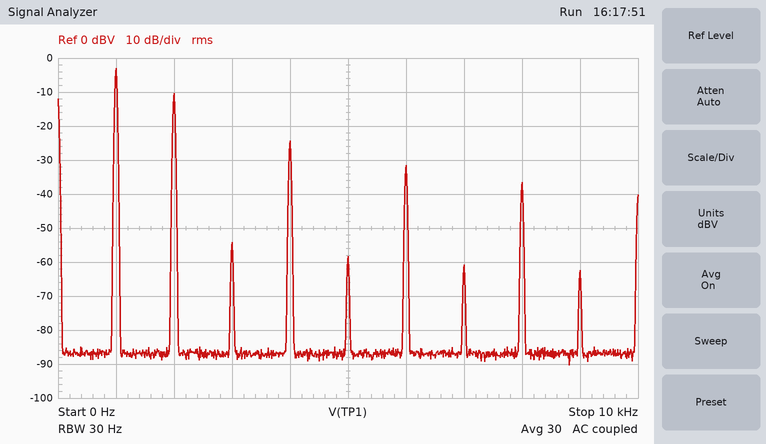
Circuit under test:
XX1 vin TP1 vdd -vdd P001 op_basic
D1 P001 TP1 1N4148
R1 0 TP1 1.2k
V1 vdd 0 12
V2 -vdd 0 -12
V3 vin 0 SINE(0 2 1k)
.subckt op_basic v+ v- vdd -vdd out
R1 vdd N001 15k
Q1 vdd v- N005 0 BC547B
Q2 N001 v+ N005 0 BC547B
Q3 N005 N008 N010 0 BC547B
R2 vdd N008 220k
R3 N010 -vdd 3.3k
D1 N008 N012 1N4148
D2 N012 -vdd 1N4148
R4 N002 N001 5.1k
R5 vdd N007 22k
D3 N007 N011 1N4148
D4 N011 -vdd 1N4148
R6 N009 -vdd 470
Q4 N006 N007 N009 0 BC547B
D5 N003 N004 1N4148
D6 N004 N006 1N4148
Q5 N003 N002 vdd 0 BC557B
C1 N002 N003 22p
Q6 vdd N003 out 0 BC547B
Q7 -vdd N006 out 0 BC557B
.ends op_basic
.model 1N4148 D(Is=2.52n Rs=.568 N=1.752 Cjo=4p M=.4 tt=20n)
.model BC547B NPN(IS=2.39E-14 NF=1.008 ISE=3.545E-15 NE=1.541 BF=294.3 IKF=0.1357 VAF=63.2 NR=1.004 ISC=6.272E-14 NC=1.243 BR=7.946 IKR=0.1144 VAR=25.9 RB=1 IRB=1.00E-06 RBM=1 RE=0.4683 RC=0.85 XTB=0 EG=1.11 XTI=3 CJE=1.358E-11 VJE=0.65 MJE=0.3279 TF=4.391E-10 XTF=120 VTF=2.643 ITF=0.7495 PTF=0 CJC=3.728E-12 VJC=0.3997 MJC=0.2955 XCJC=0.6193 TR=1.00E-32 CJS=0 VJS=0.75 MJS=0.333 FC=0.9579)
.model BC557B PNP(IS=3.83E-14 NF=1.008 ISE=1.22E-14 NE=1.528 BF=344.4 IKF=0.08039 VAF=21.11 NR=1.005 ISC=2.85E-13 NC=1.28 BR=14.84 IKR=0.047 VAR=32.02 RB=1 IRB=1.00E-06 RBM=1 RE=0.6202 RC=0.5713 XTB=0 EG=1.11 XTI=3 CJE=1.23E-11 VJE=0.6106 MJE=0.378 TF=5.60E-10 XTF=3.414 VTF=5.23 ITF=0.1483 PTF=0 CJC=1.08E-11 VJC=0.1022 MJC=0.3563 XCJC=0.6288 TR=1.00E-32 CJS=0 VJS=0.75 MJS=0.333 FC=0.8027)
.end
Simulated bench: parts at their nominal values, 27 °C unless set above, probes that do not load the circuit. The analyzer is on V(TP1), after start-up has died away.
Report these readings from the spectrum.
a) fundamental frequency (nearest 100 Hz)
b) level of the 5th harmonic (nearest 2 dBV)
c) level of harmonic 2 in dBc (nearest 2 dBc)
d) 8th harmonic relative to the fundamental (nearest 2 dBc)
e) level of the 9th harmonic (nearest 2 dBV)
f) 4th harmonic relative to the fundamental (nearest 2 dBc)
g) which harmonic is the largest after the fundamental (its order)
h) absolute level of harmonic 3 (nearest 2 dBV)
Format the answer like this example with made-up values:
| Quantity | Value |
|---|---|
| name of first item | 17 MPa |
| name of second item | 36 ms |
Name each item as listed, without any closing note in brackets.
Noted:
| Quantity | Value |
|---|---|
| fundamental frequency | 1.0 kHz |
| level of the 5th harmonic | -58 dBV |
| level of harmonic 2 in dBc | -8 dBc |
| 8th harmonic relative to the fundamental | -34 dBc |
| level of the 9th harmonic | -62 dBV |
| 4th harmonic relative to the fundamental | -22 dBc |
| which harmonic is the largest after the fundamental | 2 |
| absolute level of harmonic 3 | -54 dBV |
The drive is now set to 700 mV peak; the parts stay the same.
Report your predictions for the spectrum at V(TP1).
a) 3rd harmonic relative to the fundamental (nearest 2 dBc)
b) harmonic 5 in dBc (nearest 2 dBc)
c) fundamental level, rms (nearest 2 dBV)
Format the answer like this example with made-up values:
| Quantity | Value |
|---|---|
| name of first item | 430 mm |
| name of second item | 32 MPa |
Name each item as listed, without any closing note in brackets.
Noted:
| Quantity | Value |
|---|---|
| 3rd harmonic relative to the fundamental | -42 dBc |
| harmonic 5 in dBc | -46 dBc |
| fundamental level, rms | -12 dBV |
